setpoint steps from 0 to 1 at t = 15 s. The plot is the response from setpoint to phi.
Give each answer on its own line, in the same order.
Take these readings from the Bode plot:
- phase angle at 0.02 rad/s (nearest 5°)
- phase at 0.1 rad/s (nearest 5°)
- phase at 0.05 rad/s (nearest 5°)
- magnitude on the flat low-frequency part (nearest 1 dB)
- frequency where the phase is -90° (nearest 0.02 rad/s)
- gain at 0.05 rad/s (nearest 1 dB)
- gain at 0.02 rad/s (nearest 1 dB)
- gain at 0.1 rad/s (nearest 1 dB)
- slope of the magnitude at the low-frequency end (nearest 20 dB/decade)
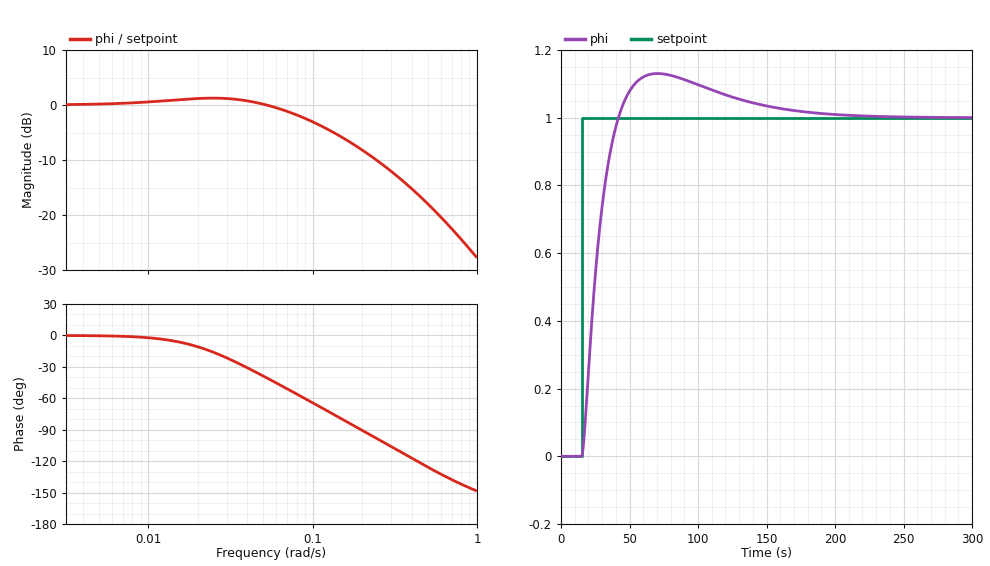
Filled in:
-10°
-65°
-40°
0 dB
0.20 rad/s
0 dB
1 dB
-3 dB
0 dB/decade
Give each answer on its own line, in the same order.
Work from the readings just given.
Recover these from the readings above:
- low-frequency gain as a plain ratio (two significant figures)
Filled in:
1.0
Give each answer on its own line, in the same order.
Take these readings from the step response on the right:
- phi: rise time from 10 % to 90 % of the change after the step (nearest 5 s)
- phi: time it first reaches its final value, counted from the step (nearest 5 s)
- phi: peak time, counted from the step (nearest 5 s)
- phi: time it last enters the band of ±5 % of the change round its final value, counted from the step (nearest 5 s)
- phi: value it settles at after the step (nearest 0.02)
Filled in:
20 s
25 s
55 s
120 s
1.00
